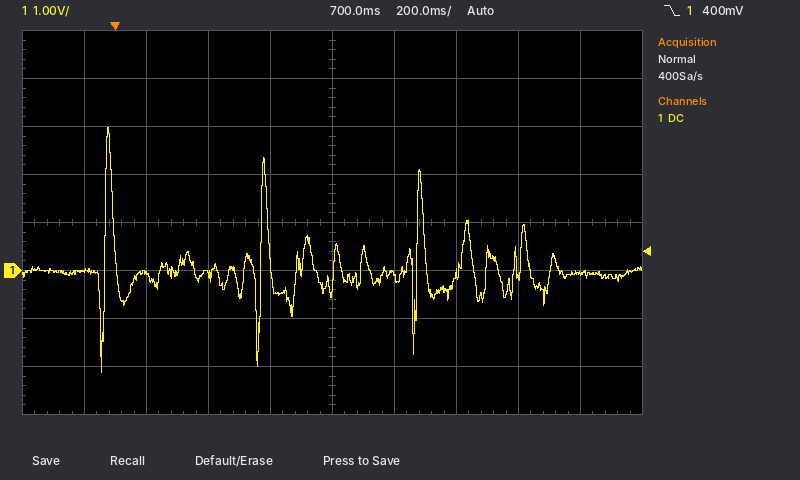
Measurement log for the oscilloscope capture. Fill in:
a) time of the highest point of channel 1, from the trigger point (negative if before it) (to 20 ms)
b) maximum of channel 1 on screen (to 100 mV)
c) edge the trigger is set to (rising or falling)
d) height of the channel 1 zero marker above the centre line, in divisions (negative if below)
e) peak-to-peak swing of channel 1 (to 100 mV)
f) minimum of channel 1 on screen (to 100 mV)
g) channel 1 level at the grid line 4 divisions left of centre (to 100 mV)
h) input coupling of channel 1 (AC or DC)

-20 ms
3.0 V
falling
-1.0 div
5.1 V
-2.1 V
0.0 V
DC
